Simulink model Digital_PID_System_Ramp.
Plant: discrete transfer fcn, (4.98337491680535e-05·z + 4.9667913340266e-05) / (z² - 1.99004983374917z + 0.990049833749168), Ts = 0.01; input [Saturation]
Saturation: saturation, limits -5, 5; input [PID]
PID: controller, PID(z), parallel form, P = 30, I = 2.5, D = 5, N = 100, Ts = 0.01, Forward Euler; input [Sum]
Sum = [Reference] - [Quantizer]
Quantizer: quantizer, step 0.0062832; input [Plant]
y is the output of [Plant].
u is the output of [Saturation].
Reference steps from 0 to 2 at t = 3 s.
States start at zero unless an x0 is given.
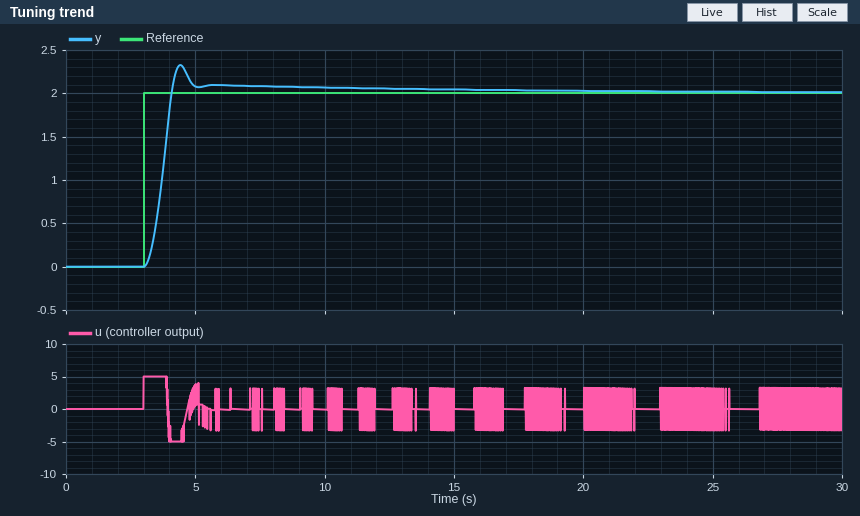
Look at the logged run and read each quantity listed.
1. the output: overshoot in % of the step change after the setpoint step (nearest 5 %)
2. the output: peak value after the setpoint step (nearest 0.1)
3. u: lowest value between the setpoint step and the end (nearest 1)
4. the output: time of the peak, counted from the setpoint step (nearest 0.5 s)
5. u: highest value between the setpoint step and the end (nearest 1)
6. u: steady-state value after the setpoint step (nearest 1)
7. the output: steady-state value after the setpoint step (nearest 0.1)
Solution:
15 %
2.3
-5
1.5 s
5
0
2.0
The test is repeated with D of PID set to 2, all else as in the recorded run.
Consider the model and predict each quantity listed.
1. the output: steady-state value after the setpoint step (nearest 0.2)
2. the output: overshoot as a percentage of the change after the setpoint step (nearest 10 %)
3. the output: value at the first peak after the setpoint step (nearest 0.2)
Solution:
2.0
30 %
2.6
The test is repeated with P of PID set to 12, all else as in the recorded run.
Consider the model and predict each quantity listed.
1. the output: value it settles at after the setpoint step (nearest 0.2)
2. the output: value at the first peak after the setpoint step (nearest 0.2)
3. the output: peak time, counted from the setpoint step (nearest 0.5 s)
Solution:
2.0
2.2
2.0 s
